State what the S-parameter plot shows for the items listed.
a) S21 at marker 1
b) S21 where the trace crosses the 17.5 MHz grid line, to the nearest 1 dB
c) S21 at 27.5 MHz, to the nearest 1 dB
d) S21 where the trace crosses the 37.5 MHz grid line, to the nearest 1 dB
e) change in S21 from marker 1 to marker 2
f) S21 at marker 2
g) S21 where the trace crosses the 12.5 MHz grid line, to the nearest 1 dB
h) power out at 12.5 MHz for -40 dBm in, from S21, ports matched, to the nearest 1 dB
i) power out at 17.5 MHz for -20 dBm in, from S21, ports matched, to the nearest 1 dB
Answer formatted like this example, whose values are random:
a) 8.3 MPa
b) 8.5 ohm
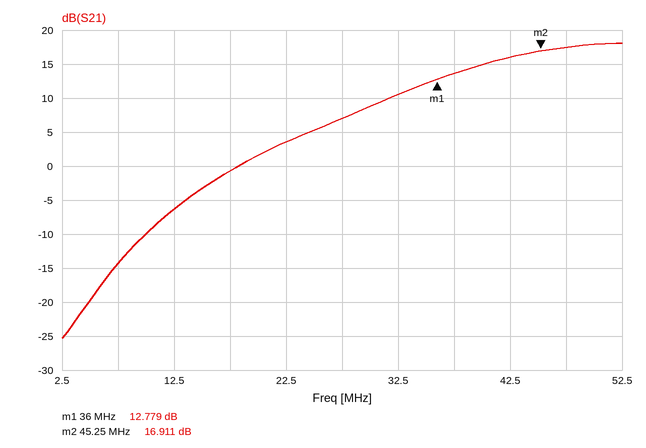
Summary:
a) 12.779 dB
b) -1 dB
c) 7 dB
d) 14 dB
e) 4.132 dB
f) 16.911 dB
g) -6 dB
h) -46 dBm
i) -21 dBm
